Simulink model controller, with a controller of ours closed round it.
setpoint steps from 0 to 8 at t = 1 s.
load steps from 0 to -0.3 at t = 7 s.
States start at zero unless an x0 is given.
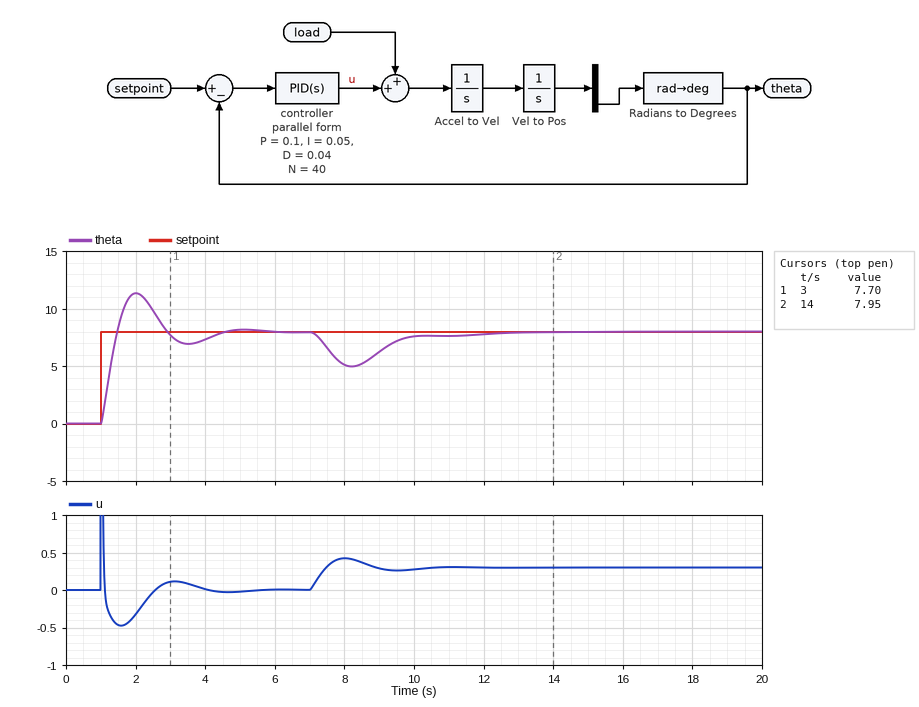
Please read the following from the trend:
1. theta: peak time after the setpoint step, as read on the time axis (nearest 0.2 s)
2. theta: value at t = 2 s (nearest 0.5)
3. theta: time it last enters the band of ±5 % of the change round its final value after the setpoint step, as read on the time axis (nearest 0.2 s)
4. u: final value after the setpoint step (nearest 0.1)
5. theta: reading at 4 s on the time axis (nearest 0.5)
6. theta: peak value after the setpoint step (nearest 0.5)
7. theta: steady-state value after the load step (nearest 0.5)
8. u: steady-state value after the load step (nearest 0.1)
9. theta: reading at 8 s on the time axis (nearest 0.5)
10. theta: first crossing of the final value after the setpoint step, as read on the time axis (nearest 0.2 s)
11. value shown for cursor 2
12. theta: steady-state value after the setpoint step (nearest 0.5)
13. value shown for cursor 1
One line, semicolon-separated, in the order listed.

2.0 s; 11.5; 4.2 s; 0.0; 7.5; 11.5; 8.0; 0.3; 5.0; 1.4 s; 7.95; 8.0; 7.70
